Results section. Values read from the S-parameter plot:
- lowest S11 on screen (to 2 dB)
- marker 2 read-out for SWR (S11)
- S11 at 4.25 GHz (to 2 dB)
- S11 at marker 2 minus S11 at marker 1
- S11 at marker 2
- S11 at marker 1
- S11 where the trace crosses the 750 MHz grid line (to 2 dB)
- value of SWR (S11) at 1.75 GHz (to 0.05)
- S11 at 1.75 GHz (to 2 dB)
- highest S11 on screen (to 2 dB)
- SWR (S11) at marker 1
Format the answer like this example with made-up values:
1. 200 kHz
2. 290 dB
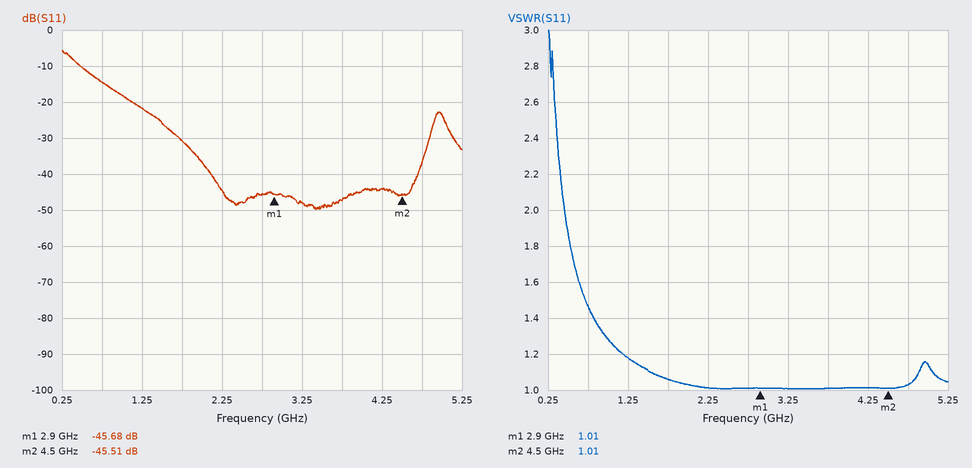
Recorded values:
1. -50 dB
2. 1.01
3. -44 dB
4. 0.17 dB
5. -45.51 dB
6. -45.68 dB
7. -14 dB
8. 1.05
9. -30 dB
10. -6 dB
11. 1.01
